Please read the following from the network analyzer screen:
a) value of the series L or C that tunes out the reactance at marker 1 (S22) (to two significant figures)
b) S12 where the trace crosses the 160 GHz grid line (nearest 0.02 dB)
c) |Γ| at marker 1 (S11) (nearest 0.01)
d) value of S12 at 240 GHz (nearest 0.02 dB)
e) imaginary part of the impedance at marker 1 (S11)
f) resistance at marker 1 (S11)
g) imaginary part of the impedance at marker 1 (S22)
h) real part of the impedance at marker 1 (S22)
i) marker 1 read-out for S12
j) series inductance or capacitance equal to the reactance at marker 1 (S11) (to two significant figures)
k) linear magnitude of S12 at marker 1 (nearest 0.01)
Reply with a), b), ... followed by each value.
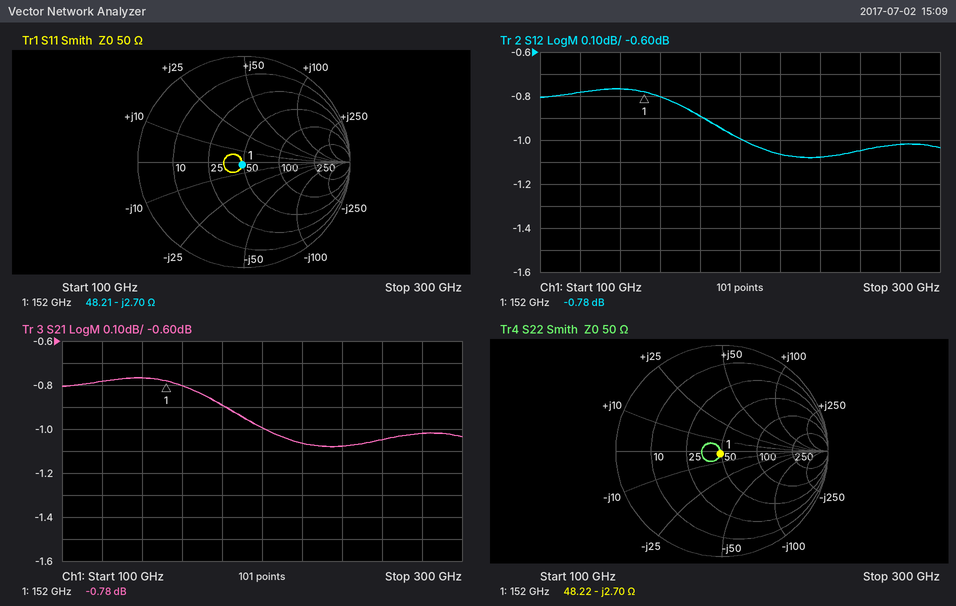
a) 2.8 pH
b) -0.80 dB
c) 0.03
d) -1.08 dB
e) -2.70 Ω
f) 48.21 Ω
g) -2.70 Ω
h) 48.22 Ω
i) -0.78 dB
j) 390 fF
k) 0.91
